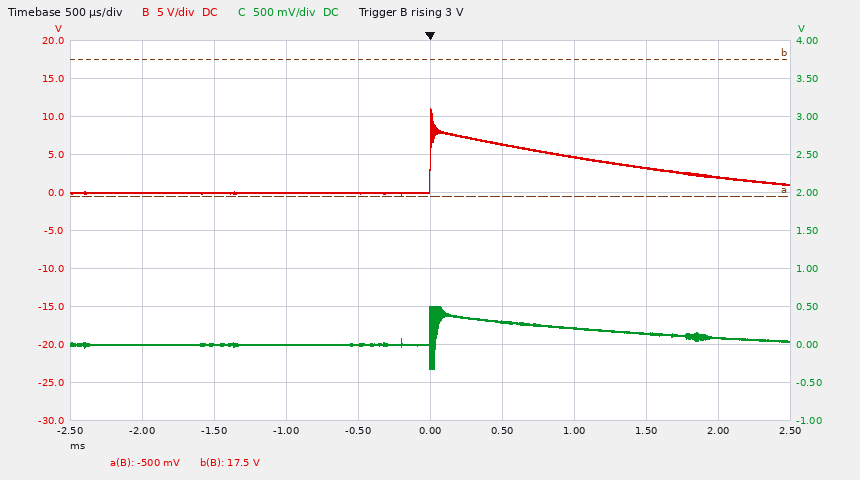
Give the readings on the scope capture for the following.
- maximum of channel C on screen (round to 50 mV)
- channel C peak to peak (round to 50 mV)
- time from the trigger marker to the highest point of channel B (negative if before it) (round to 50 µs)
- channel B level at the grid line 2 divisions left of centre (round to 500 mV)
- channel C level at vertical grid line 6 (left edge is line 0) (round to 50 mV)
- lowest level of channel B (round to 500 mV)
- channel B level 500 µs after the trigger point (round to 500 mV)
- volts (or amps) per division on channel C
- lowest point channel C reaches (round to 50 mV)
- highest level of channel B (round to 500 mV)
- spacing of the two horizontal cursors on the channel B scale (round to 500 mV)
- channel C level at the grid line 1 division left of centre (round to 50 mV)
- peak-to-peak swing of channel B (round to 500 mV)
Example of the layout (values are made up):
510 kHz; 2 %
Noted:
500 mV; 800 mV; 0 µs; 0.0 V; 300 mV; -500 mV; 6.5 V; 500 mV; -300 mV; 11.0 V; 18.0 V; 0 mV; 11.5 V
